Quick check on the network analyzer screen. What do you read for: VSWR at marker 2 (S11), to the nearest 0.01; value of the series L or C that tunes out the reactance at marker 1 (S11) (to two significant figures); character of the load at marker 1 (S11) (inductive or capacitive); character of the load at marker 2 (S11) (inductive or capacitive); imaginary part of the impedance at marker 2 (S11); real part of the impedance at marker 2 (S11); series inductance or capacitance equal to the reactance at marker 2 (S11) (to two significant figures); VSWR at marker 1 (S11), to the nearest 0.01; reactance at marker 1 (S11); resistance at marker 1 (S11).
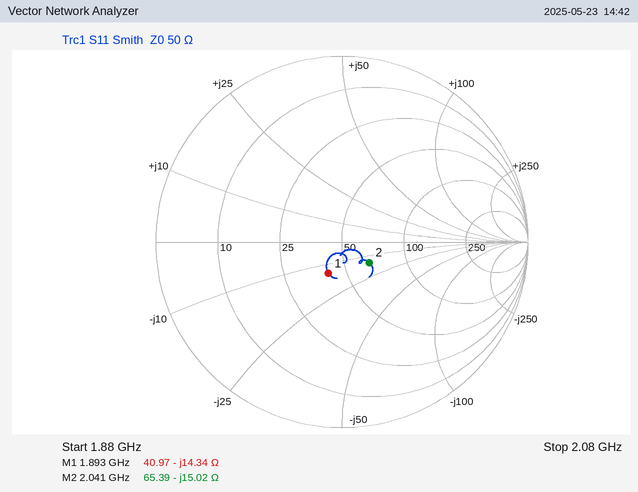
1.45
1.2 nH
capacitive
capacitive
-15.02 Ω
65.39 Ω
5.2 pF
1.45
-14.34 Ω
40.97 Ω
